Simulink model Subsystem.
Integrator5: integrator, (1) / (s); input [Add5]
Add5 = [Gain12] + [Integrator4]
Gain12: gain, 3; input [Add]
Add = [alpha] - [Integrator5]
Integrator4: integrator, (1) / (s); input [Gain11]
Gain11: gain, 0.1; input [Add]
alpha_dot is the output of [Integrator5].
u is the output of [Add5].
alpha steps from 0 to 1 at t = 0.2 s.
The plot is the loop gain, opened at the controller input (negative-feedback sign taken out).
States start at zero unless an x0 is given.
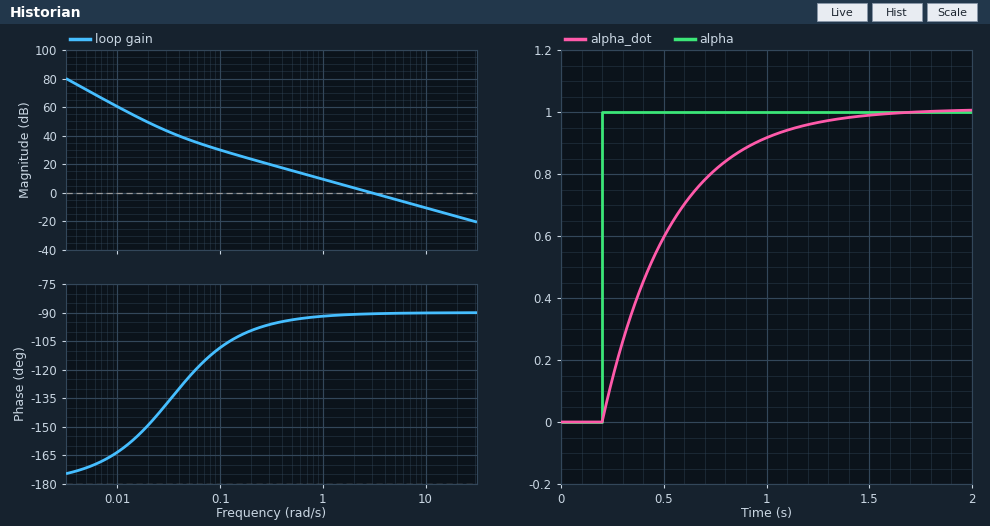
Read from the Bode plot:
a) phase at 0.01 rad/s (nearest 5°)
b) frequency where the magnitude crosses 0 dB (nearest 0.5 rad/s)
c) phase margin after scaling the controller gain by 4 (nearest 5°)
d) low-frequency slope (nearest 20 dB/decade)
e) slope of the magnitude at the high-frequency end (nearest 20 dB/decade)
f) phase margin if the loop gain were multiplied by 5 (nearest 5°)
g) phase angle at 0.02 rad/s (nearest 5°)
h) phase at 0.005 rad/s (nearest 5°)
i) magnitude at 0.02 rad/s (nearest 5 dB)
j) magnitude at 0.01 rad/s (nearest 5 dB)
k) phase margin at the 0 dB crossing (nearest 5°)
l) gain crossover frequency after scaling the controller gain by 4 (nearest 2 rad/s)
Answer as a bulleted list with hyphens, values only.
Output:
- -165°
- 3.0 rad/s
- 90°
- -40 dB/decade
- -20 dB/decade
- 90°
- -150°
- -170°
- 50 dB
- 60 dB
- 90°
- 12 rad/s
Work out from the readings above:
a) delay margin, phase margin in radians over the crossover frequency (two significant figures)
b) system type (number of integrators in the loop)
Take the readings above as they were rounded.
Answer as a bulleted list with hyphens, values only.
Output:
- 0.52 s
- 2
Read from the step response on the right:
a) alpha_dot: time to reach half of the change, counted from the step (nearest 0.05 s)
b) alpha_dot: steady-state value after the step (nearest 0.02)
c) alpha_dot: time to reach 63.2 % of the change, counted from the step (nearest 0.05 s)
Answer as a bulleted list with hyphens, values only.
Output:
- 0.25 s
- 1.00
- 0.35 s
